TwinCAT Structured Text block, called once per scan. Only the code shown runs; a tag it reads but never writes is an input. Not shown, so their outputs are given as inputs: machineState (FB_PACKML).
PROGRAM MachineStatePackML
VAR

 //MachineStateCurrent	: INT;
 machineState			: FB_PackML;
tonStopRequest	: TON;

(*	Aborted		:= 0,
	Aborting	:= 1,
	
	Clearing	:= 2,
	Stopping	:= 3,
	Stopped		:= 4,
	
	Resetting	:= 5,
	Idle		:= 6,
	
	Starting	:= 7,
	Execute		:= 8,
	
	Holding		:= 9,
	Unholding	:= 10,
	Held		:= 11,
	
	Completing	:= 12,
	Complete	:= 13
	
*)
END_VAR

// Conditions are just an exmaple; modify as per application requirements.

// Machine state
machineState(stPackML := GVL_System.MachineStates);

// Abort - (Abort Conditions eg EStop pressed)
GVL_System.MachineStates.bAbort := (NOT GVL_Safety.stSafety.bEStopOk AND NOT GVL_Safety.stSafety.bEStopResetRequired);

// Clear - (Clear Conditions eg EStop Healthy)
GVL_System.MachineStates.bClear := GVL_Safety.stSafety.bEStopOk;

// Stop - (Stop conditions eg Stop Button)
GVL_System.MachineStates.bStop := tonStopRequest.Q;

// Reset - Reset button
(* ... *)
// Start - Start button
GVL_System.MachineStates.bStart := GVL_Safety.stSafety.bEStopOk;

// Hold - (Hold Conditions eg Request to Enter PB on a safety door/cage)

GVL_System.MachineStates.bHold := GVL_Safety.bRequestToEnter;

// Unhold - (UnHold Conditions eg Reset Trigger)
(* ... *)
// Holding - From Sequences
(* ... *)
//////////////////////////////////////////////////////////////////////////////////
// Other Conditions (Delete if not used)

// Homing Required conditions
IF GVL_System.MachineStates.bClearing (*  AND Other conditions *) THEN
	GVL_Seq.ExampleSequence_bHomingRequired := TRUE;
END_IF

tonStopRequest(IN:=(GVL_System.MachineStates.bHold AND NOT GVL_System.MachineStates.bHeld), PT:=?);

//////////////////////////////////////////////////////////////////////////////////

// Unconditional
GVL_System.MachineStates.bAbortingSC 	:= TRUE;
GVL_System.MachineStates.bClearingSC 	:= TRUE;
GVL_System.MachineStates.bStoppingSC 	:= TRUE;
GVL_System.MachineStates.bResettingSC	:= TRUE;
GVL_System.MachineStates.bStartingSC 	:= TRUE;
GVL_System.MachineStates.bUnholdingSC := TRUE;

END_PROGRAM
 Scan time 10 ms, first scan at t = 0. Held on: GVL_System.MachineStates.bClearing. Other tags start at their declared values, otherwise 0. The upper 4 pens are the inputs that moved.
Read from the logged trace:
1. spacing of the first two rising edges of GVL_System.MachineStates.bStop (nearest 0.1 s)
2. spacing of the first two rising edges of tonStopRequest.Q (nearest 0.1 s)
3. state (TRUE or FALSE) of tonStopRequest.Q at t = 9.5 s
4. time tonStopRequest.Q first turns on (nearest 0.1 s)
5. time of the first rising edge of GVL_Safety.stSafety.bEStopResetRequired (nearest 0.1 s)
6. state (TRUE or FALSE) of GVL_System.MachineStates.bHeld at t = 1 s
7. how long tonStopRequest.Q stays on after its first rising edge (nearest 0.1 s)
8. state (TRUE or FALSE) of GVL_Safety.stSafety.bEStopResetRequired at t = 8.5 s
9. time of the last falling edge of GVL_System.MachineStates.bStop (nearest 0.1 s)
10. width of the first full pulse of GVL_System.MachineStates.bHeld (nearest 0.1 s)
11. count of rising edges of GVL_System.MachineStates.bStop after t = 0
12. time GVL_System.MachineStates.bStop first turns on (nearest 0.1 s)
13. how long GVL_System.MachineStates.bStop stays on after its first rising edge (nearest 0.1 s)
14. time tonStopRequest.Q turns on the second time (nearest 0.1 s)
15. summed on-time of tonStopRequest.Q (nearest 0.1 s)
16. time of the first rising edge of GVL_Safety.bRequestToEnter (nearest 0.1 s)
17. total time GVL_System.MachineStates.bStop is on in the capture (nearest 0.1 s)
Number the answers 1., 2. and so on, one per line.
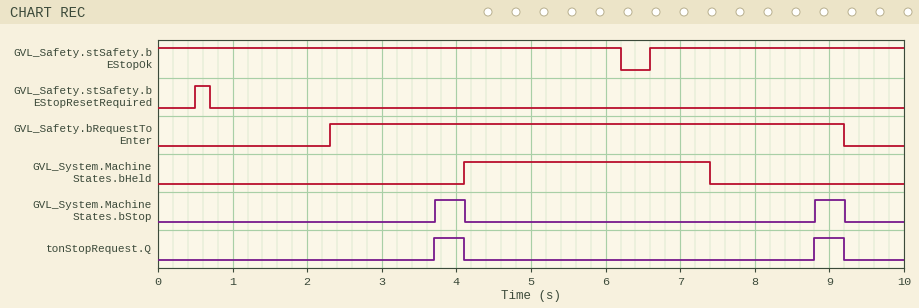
1. 5.1 s
2. 5.1 s
3. FALSE
4. 3.7 s
5. 0.5 s
6. FALSE
7. 0.4 s
8. FALSE
9. 9.2 s
10. 3.3 s
11. 2
12. 3.7 s
13. 0.4 s
14. 8.8 s
15. 0.8 s
16. 2.3 s
17. 0.8 s
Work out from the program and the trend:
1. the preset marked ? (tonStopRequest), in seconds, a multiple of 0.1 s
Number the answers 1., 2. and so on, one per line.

1. 1.4 s
